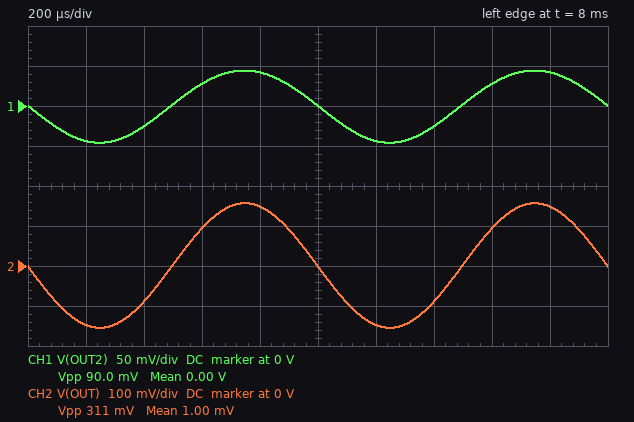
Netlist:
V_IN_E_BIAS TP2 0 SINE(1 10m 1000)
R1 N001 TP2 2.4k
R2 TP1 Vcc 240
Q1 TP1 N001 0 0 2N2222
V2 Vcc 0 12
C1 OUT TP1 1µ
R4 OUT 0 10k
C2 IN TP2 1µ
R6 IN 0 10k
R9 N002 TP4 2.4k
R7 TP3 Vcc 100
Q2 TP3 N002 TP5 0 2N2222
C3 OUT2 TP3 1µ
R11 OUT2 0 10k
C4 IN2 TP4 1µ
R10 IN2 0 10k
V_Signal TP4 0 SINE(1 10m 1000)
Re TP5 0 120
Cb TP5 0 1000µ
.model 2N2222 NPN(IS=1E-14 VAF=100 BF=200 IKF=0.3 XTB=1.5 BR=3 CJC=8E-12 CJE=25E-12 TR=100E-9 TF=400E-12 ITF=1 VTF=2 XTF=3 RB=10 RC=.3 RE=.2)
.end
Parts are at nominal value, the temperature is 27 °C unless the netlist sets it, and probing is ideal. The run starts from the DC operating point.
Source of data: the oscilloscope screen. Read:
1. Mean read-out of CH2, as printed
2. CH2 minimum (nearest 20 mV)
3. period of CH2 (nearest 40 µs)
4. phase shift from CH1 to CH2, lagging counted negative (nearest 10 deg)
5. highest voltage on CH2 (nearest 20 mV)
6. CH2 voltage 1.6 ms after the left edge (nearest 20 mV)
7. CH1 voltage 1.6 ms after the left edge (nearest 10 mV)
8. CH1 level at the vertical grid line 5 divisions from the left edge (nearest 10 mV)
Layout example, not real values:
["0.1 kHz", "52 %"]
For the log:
["1.00 mV", "-160 mV", "1.00 ms", "0 deg", "160 mV", "100 mV", "30 mV", "0 V"]
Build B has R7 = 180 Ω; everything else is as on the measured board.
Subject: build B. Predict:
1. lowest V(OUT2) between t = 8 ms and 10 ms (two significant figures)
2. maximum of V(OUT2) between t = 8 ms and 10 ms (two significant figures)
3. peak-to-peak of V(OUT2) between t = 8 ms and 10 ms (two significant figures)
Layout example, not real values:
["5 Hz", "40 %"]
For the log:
["-82 mV", "79 mV", "160 mV"]
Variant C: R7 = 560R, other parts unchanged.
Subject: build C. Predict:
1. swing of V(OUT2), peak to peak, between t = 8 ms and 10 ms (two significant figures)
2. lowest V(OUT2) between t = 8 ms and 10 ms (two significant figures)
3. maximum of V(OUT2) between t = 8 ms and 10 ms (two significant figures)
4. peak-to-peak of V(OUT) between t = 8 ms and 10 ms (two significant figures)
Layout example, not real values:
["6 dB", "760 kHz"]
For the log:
["480 mV", "-240 mV", "230 mV", "310 mV"]
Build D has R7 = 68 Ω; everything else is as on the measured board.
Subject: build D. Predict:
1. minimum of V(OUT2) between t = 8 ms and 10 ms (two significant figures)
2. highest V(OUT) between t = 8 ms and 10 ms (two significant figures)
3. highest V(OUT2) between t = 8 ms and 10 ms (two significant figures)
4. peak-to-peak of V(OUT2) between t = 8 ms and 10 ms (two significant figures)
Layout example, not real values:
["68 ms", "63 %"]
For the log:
["-31 mV", "160 mV", "30 mV", "62 mV"]
